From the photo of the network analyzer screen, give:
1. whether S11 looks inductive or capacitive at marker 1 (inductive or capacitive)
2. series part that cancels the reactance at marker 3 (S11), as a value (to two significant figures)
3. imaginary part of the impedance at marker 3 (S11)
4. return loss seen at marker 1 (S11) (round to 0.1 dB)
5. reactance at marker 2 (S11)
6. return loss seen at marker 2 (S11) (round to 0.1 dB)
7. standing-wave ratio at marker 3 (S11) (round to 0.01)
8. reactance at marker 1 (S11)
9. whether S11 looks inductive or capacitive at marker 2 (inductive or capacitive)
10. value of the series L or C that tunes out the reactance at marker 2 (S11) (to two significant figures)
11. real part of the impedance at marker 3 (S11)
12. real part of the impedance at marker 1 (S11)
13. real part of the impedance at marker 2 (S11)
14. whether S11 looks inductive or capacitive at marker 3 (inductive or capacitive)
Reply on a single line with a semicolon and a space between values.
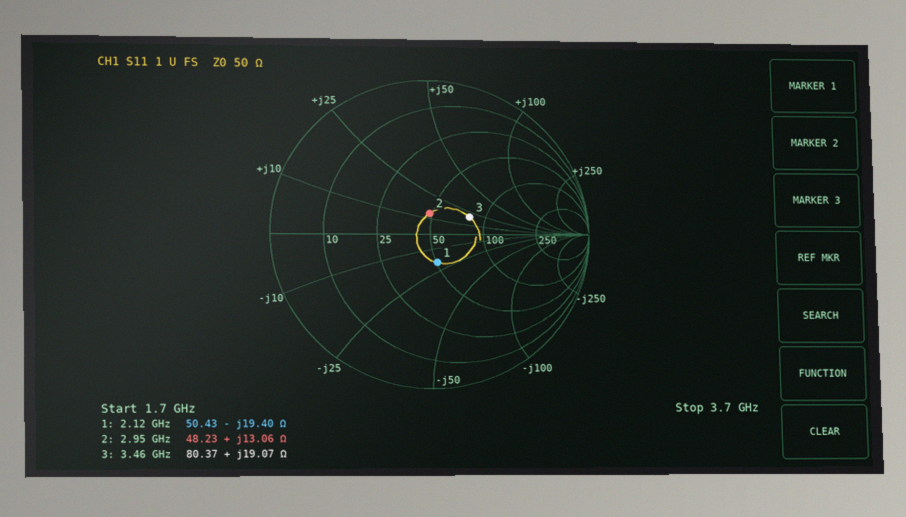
capacitive; 2.4 pF; +19.07 Ω; 14.4 dB; +13.06 Ω; 17.5 dB; 1.75; -19.40 Ω; inductive; 4.1 pF; 80.37 Ω; 50.43 Ω; 48.23 Ω; inductive
